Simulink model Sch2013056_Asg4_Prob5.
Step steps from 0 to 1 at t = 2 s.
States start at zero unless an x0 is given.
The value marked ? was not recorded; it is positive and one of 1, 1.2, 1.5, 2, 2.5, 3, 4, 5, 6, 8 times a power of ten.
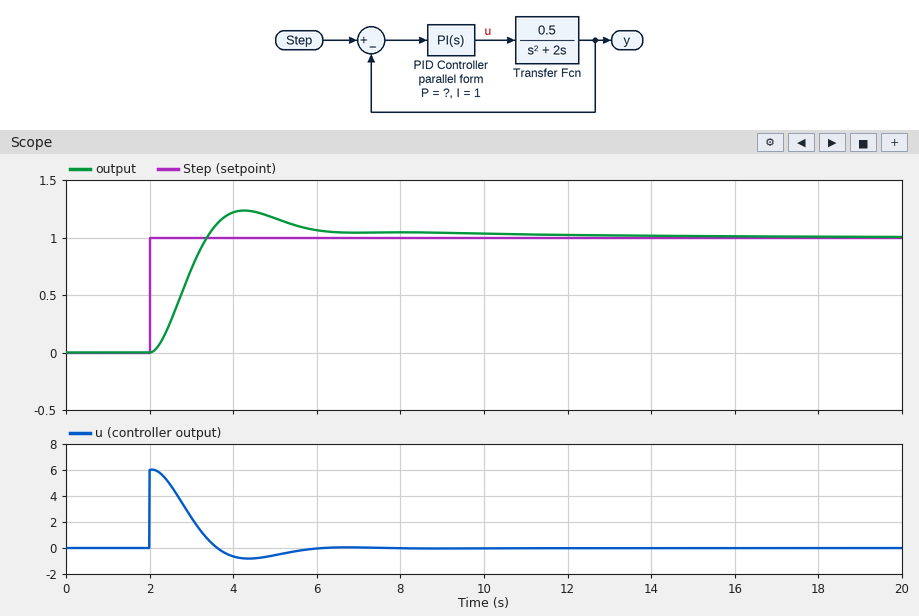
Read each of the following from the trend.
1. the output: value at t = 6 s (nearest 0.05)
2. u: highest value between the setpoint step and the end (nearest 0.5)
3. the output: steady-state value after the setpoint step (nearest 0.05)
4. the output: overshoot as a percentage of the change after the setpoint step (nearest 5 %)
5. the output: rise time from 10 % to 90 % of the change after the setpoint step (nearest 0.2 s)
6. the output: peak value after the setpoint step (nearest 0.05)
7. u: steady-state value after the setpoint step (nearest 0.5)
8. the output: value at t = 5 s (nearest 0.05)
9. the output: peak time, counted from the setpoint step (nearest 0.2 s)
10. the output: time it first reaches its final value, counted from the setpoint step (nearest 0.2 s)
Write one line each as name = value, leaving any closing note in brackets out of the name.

the output: value at t = 6 s = 1.05
u: highest value between the setpoint step and the end = 6.0
the output: steady-state value after the setpoint step = 1.00
the output: overshoot as a percentage of the change after the setpoint step = 25 %
the output: rise time from 10 % to 90 % of the change after the setpoint step = 1.0 s
the output: peak value after the setpoint step = 1.25
u: steady-state value after the setpoint step = 0.0
the output: value at t = 5 s = 1.15
the output: peak time, counted from the setpoint step = 2.2 s
the output: time it first reaches its final value, counted from the setpoint step = 1.4 s
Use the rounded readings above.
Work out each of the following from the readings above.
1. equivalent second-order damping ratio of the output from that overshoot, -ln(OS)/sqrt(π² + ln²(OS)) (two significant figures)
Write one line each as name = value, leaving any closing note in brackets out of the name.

equivalent second-order damping ratio of the output from that overshoot, -ln(OS)/sqrt(π² + ln²(OS)) = 0.40
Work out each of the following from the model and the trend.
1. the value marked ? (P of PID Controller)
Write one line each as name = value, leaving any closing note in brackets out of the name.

the value marked ? = 6
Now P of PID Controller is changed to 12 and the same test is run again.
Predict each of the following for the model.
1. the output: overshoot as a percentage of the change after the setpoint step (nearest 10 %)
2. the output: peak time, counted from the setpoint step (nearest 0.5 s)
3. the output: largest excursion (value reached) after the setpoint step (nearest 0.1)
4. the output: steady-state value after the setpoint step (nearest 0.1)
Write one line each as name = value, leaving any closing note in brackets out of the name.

the output: overshoot as a percentage of the change after the setpoint step = 30 %
the output: peak time, counted from the setpoint step = 1.5 s
the output: largest excursion (value reached) after the setpoint step = 1.3
the output: steady-state value after the setpoint step = 1.0
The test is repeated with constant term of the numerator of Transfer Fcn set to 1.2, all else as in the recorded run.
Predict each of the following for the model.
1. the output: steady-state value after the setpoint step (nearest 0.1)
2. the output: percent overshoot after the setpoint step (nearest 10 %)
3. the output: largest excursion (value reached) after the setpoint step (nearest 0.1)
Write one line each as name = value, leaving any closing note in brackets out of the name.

the output: steady-state value after the setpoint step = 1.0
the output: percent overshoot after the setpoint step = 40 %
the output: largest excursion (value reached) after the setpoint step = 1.4
